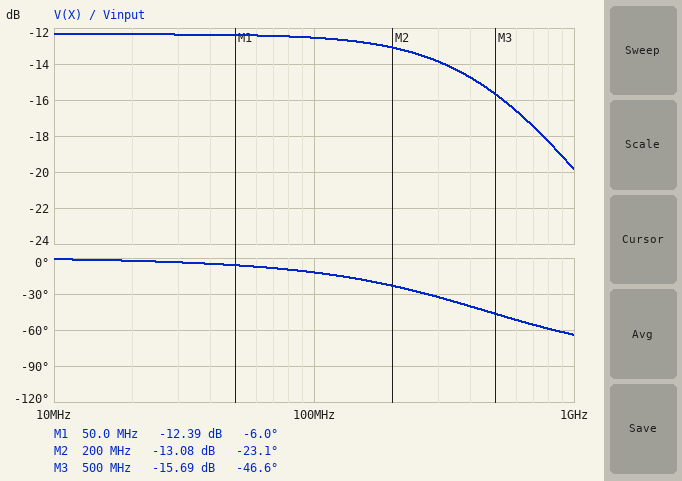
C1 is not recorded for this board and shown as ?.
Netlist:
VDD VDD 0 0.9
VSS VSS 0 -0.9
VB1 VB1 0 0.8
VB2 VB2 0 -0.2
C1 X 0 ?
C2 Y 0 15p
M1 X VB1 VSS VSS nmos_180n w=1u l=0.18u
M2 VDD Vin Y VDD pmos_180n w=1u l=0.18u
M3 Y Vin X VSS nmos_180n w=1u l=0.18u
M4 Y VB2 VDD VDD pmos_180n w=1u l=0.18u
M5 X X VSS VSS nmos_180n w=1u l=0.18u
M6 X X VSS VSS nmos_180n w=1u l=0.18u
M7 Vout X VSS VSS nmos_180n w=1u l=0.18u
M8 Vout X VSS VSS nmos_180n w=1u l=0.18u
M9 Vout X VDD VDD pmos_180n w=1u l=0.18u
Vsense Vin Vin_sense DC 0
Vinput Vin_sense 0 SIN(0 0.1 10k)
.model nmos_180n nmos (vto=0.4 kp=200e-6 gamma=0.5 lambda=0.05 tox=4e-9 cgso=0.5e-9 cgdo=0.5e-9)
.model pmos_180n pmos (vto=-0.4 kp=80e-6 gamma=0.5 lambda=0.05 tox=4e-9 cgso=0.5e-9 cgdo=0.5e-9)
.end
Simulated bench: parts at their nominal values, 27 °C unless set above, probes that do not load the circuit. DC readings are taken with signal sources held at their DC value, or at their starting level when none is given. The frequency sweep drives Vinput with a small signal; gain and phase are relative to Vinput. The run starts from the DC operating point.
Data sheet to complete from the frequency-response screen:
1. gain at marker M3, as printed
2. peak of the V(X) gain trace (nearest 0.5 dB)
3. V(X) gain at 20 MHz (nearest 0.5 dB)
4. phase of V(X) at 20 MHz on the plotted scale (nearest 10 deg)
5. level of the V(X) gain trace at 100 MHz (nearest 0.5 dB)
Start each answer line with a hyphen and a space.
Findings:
- -15.69 dB
- -12.5 dB
- -12.5 dB
- 0 deg
- -12.5 dB
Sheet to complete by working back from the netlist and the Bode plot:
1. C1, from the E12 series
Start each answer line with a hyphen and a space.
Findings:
- 680 fF
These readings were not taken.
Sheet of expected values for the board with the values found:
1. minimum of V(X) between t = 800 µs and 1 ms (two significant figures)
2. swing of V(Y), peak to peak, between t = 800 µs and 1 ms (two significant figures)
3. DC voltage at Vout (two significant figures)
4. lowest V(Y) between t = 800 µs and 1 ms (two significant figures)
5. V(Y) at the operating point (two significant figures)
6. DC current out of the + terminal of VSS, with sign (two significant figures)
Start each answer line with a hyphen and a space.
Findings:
- -850 mV
- 320 mV
- 900 mV
- 450 mV
- 670 mV
- -99 µA
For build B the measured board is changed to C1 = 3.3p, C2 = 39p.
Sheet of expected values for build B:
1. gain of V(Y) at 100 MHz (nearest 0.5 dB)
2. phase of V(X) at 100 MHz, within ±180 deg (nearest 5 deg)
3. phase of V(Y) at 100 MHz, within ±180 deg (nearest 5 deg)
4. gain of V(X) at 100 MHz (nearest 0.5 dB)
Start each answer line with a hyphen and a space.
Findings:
- -33.5 dB
- -45 deg
- 100 deg
- -15.5 dB
